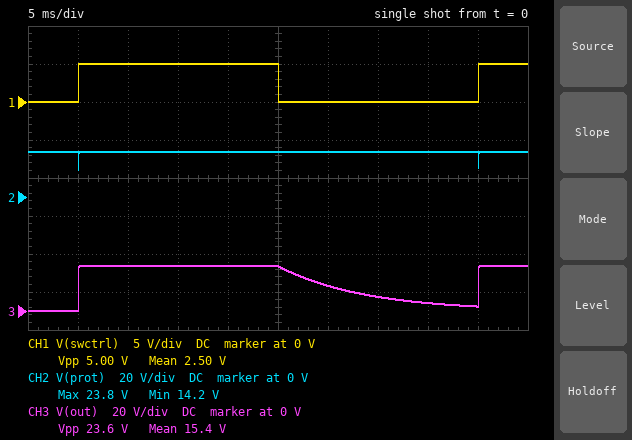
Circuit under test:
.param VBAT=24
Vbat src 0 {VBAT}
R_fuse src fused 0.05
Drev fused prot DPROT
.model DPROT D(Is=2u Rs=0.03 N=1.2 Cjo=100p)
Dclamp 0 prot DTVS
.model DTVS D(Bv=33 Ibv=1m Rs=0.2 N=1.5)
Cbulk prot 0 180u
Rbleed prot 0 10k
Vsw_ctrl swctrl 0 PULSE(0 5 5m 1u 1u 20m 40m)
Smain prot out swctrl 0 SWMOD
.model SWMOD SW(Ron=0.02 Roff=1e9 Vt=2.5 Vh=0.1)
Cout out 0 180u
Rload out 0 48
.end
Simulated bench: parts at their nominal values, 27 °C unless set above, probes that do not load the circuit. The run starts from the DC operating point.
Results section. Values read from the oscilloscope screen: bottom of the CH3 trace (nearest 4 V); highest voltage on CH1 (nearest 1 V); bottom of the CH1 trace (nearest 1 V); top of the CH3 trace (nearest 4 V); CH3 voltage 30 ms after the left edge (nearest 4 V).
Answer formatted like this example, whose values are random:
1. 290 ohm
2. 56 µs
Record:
1. 0 V
2. 5 V
3. 0 V
4. 24 V
5. 12 V
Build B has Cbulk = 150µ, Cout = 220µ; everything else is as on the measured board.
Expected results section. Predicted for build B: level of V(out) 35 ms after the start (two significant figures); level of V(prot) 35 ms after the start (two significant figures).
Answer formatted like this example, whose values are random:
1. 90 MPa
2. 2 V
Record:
1. 9.1 V
2. 24 V
